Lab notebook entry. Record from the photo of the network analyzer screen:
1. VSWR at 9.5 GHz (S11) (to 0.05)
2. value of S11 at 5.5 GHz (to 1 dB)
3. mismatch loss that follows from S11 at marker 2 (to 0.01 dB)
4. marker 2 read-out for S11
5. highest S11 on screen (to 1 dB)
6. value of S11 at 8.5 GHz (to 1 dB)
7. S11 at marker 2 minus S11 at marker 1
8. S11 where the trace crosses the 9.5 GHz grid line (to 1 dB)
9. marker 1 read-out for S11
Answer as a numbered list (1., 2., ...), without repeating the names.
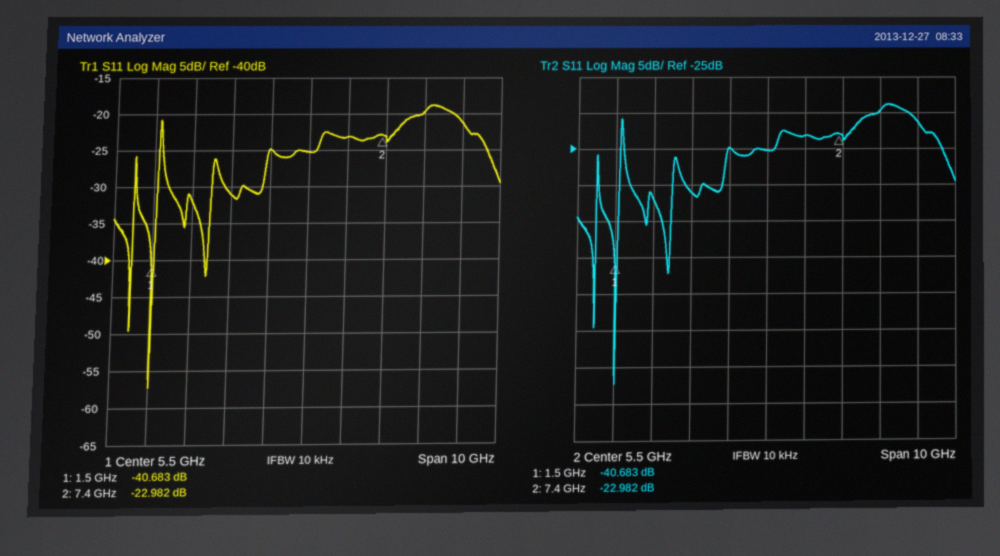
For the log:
1. 1.20
2. -25 dB
3. 0.02 dB
4. -22.982 dB
5. -19 dB
6. -20 dB
7. 17.701 dB
8. -21 dB
9. -40.683 dB
